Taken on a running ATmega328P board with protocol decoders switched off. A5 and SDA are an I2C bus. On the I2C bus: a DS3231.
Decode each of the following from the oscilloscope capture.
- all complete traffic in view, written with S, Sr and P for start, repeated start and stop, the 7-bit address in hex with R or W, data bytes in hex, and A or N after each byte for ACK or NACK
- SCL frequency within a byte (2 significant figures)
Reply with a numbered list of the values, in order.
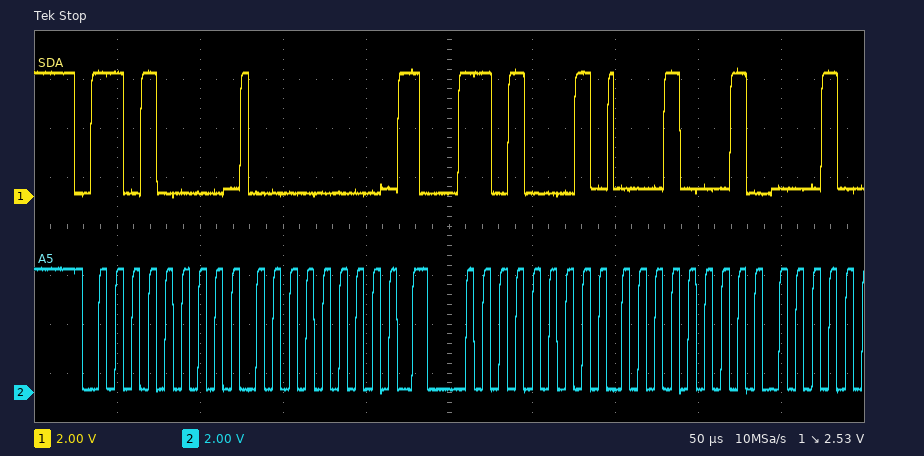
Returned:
1. S 68W A 00 A Sr 68R A 11 A
2. 100 kHz
